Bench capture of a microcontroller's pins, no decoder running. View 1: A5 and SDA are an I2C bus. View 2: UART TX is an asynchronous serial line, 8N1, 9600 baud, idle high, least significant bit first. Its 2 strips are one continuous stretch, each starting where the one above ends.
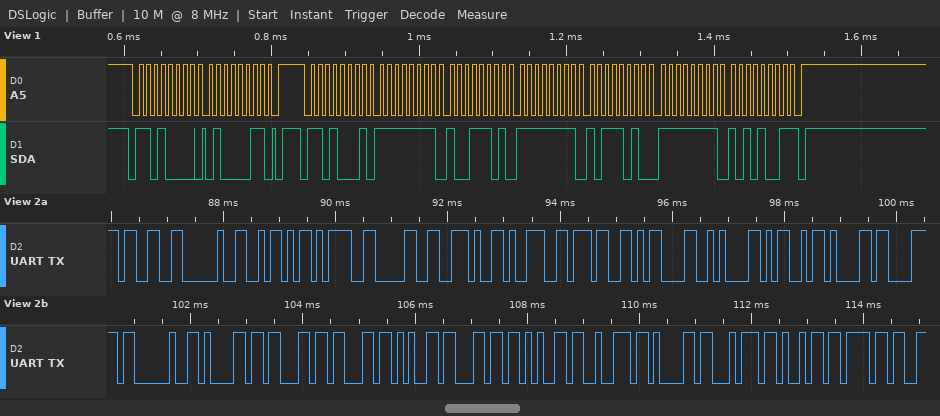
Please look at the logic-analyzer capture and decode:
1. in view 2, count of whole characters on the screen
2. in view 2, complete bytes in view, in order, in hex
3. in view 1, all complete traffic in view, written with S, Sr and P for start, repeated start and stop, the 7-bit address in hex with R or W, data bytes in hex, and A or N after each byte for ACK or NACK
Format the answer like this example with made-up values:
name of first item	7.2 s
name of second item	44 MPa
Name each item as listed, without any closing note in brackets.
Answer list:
in view 2, count of whole characters on the screen	25
in view 2, complete bytes in view, in order, in hex	0x33 0x20 0x5A 0x3D 0x30 0x2E 0x39 0x37 0x0D 0x0A 0x4D 0x61 0x78 0x20 0x61 0x63 0x63 0x65 0x6C 0x65 0x72 0x61 0x74 0x69 0x6F
in view 1, all complete traffic in view, written with S, Sr and P for start, repeated start and stop, the 7-bit address in hex with R or W, data bytes in hex, and A or N after each byte for ACK or NACK	S 68W A 43 A P S 68R A FF A 9D A FF A BA A FF A A9 N P
